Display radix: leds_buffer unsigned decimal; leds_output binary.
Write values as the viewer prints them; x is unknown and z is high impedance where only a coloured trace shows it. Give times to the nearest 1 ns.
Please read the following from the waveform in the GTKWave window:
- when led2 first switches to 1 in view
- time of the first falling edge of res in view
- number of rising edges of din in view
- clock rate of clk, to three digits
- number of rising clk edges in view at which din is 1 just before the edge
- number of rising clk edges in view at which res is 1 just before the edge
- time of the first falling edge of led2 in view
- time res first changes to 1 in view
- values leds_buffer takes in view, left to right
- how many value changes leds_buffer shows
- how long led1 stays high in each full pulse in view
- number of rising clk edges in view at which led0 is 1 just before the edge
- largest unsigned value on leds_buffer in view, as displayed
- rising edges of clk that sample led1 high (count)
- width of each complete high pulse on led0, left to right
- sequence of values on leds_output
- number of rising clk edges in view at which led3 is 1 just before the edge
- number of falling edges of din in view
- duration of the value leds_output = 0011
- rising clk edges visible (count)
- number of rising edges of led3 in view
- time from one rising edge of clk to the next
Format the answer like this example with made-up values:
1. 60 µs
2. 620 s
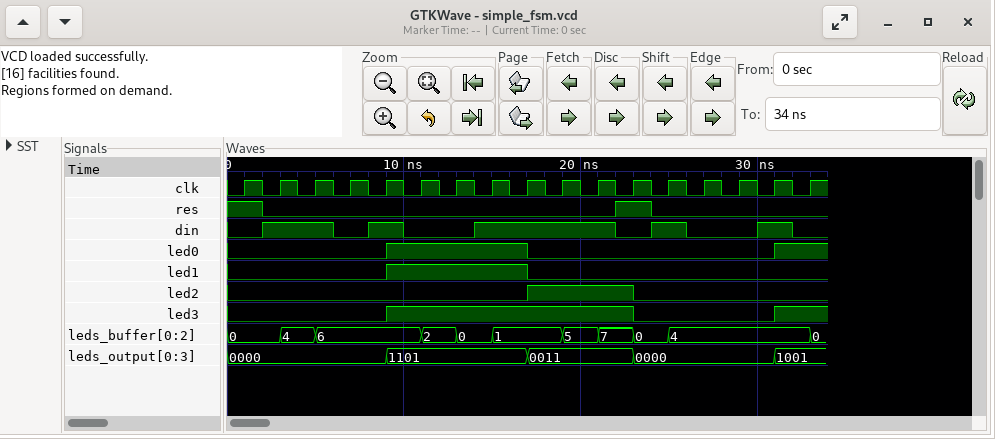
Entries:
1. 17 ns
2. 2 ns
3. 5
4. 500 MHz
5. 9
6. 2
7. 23 ns
8. 22 ns
9. 0, 4, 6, 2, 0, 1, 5, 7, 0, 4, 0
10. 10
11. 8 ns
12. 5
13. 7
14. 4
15. 8 ns
16. 0000, 1101, 0011, 0000, 1001
17. 8
18. 5
19. 6 ns
20. 17
21. 2
22. 2 ns
